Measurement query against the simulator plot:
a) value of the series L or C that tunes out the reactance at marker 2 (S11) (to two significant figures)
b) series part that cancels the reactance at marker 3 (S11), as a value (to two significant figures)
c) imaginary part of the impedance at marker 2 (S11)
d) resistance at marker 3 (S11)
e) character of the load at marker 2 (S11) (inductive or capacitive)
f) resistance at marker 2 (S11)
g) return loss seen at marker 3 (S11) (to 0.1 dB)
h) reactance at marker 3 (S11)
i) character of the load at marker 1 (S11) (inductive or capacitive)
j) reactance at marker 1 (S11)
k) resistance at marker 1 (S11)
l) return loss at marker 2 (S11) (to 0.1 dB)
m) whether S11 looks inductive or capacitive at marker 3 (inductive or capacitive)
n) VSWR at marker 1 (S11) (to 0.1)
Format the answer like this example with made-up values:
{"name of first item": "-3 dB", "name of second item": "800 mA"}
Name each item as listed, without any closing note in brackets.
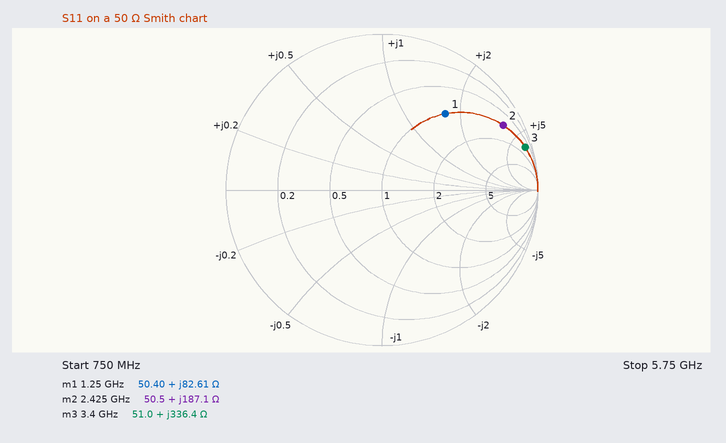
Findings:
{"value of the series L or C that tunes out the reactance at marker 2 (S11)": "350 fF", "series part that cancels the reactance at marker 3 (S11), as a value": "140 fF", "imaginary part of the impedance at marker 2": "+187.1 Ω", "resistance at marker 3": "51.0 Ω", "character of the load at marker 2 (S11)": "inductive", "resistance at marker 2": "50.5 Ω", "return loss seen at marker 3 (S11)": "0.4 dB", "reactance at marker 3": "+336.4 Ω", "character of the load at marker 1 (S11)": "inductive", "reactance at marker 1": "+82.61 Ω", "resistance at marker 1": "50.40 Ω", "return loss at marker 2 (S11)": "1.1 dB", "whether S11 looks inductive or capacitive at marker 3": "inductive", "VSWR at marker 1 (S11)": "4.5"}
